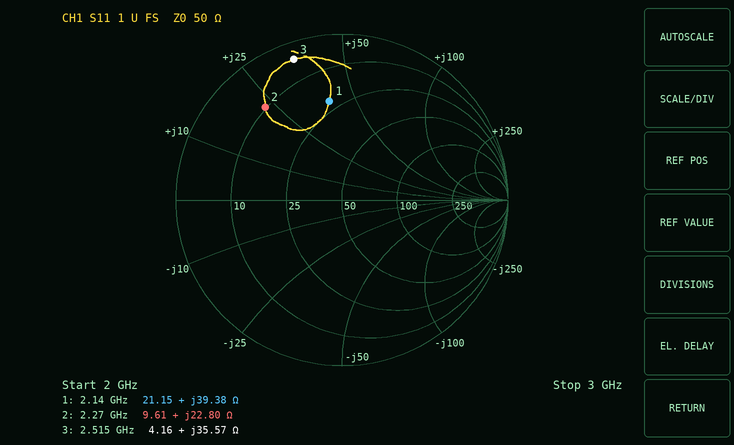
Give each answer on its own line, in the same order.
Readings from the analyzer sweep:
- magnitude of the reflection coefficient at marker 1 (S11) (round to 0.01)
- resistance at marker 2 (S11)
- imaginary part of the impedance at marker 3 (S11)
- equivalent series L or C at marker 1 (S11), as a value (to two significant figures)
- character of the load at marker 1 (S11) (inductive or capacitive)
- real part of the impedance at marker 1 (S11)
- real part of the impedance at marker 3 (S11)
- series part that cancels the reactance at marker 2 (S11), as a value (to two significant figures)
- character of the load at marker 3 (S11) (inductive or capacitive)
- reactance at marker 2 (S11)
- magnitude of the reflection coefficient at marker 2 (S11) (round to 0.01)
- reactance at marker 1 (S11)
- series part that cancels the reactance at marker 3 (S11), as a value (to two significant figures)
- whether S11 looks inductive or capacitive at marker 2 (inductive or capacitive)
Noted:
0.60
9.61 Ω
+35.57 Ω
2.9 nH
inductive
21.15 Ω
4.16 Ω
3.1 pF
inductive
+22.80 Ω
0.73
+39.38 Ω
1.8 pF
inductive
